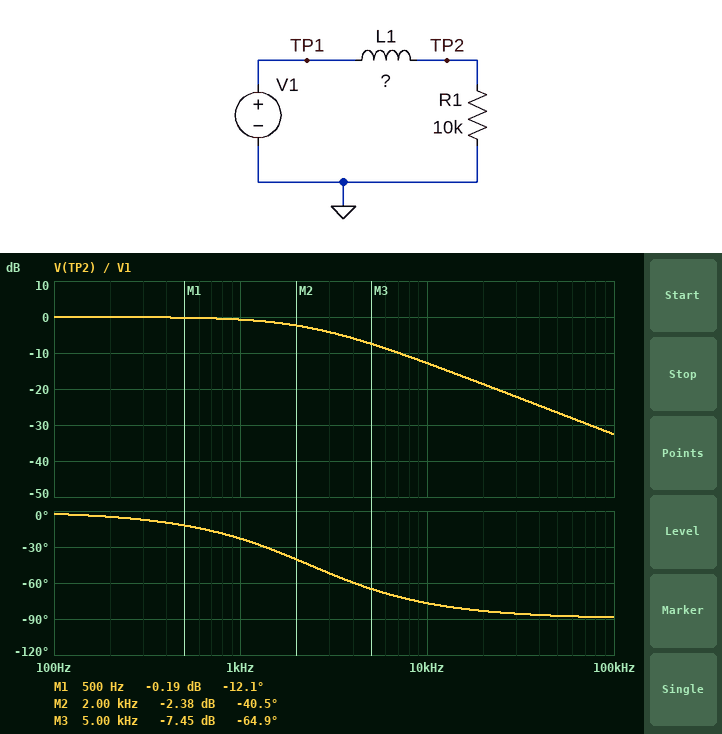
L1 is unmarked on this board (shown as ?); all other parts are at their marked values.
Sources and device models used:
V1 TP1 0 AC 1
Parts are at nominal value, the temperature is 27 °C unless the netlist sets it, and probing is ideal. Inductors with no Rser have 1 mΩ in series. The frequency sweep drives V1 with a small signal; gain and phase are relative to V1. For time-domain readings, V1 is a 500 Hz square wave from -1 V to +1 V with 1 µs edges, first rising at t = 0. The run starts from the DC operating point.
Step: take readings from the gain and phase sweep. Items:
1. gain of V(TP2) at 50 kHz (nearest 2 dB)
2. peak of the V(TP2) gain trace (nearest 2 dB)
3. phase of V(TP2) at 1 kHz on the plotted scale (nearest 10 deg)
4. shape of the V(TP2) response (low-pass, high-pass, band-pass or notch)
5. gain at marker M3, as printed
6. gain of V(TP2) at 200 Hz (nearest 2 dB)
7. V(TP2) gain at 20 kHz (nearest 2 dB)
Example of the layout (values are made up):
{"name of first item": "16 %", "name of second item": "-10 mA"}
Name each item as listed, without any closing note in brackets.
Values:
{"gain of V(TP2) at 50 kHz": "-26 dB", "peak of the V(TP2) gain trace": "0 dB", "phase of V(TP2) at 1 kHz on the plotted scale": "-20 deg", "shape of the V(TP2) response": "low-pass", "gain at marker M3, as printed": "-7.45 dB", "gain of V(TP2) at 200 Hz": "0 dB", "V(TP2) gain at 20 kHz": "-18 dB"}
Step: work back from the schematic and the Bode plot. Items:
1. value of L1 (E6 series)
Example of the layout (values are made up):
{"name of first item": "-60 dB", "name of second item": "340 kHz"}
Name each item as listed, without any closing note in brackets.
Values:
{"value of L1": "680 mH"}
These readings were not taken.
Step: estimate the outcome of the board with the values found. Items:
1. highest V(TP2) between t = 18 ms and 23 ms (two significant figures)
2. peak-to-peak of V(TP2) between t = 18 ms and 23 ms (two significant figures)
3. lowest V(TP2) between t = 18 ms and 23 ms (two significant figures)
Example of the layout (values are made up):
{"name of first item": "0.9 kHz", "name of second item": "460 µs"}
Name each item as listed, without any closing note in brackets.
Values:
{"highest V(TP2) between t = 18 ms and 23 ms": "1.0 V", "peak-to-peak of V(TP2) between t = 18 ms and 23 ms": "2.0 V", "lowest V(TP2) between t = 18 ms and 23 ms": "-1.0 V"}
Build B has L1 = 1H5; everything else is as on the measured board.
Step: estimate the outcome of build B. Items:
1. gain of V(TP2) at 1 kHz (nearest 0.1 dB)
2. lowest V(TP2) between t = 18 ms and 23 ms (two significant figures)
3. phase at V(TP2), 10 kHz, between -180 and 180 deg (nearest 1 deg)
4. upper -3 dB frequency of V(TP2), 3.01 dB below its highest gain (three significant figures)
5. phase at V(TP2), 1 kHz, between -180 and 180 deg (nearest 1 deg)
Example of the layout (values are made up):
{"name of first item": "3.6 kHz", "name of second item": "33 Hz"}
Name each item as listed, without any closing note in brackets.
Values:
{"gain of V(TP2) at 1 kHz": "-2.8 dB", "lowest V(TP2) between t = 18 ms and 23 ms": "-1.0 V", "phase at V(TP2), 10 kHz, between -180 and 180 deg": "-84 deg", "upper -3 dB frequency of V(TP2), 3.01 dB below its highest gain": "1.06 kHz", "phase at V(TP2), 1 kHz, between -180 and 180 deg": "-43 deg"}
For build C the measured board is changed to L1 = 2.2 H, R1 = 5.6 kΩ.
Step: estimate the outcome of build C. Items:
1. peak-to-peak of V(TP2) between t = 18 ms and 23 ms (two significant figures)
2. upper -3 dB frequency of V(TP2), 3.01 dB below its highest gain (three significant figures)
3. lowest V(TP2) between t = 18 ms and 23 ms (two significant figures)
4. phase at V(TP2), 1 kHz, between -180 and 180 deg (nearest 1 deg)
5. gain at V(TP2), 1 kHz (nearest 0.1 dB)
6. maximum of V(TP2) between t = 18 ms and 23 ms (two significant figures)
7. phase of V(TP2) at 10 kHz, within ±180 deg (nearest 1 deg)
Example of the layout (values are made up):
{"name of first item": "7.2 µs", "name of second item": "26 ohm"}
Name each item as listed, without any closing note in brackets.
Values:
{"peak-to-peak of V(TP2) between t = 18 ms and 23 ms": "1.7 V", "upper -3 dB frequency of V(TP2), 3.01 dB below its highest gain": "405 Hz", "lowest V(TP2) between t = 18 ms and 23 ms": "-850 mV", "phase at V(TP2), 1 kHz, between -180 and 180 deg": "-68 deg", "gain at V(TP2), 1 kHz": "-8.5 dB", "maximum of V(TP2) between t = 18 ms and 23 ms": "850 mV", "phase of V(TP2) at 10 kHz, within ±180 deg": "-88 deg"}
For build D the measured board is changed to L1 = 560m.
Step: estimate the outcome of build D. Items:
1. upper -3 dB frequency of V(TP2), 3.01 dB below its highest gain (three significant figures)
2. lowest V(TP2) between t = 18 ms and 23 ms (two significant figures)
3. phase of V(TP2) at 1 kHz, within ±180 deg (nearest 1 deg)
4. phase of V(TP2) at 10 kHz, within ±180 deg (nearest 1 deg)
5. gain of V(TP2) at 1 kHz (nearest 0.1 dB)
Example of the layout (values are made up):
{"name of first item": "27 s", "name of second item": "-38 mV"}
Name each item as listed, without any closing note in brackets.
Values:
{"upper -3 dB frequency of V(TP2), 3.01 dB below its highest gain": "2.84 kHz", "lowest V(TP2) between t = 18 ms and 23 ms": "-1.0 V", "phase of V(TP2) at 1 kHz, within ±180 deg": "-19 deg", "phase of V(TP2) at 10 kHz, within ±180 deg": "-74 deg", "gain of V(TP2) at 1 kHz": "-0.5 dB"}
